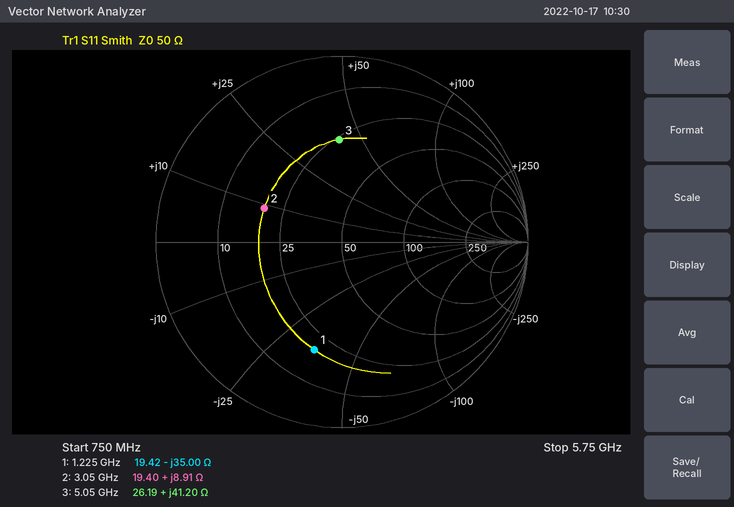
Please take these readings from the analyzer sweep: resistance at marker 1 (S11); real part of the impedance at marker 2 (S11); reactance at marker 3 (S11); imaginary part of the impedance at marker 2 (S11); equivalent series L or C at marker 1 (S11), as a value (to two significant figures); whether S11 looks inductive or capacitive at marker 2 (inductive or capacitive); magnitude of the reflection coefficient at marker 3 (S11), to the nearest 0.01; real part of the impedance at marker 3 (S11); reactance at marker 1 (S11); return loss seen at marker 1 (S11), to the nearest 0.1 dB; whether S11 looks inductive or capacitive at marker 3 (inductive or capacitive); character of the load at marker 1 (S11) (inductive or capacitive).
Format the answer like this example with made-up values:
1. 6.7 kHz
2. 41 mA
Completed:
1. 19.42 Ω
2. 19.40 Ω
3. +41.20 Ω
4. +8.91 Ω
5. 3.7 pF
6. inductive
7. 0.55
8. 26.19 Ω
9. -35.00 Ω
10. 4.5 dB
11. inductive
12. capacitive
